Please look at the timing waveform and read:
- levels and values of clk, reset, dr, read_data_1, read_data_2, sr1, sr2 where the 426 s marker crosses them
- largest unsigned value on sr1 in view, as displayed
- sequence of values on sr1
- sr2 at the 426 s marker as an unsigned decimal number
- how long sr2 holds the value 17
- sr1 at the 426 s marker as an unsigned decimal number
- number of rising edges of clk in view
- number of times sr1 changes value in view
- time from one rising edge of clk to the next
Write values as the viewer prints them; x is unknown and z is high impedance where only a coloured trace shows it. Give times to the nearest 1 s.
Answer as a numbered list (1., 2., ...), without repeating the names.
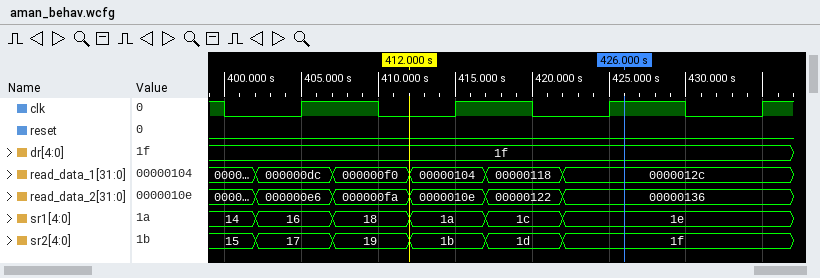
1. clk=1, reset=0, dr=1f, read_data_1=0000012c, read_data_2=00000136, sr1=1e, sr2=1f
2. 1e
3. 14, 16, 18, 1a, 1c, 1e
4. 31
5. 5 s
6. 30
7. 4
8. 5
9. 10 s
